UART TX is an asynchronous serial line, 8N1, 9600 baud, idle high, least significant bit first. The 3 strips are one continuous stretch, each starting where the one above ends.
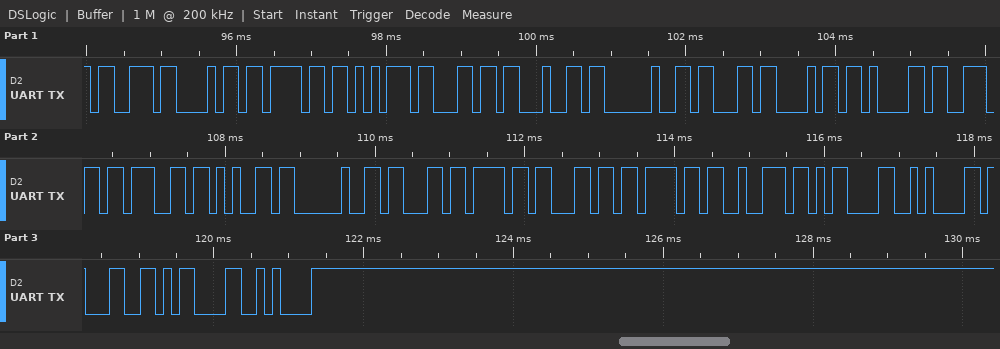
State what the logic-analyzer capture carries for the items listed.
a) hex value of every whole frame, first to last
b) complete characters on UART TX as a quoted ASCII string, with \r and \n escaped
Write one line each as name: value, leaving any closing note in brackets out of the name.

hex value of every whole frame, first to last: 0x73 0x68 0x6F 0x75 0x6C 0x64 0x20 0x63 0x68 0x61 0x6E 0x67 0x65 0x20 0x63 0x6F 0x6C 0x6F 0x72 0x0D 0x0A 0x31 0x0D 0x0A
complete characters on UART TX as a quoted ASCII string, with \r and \n escaped: "should change color\r\n1\r\n"
